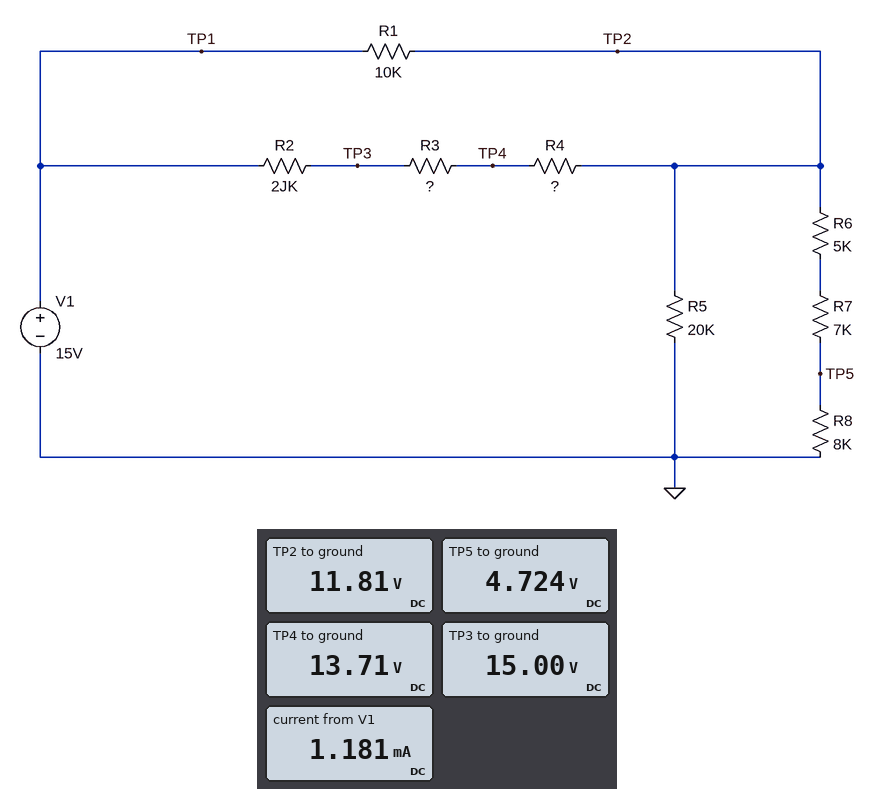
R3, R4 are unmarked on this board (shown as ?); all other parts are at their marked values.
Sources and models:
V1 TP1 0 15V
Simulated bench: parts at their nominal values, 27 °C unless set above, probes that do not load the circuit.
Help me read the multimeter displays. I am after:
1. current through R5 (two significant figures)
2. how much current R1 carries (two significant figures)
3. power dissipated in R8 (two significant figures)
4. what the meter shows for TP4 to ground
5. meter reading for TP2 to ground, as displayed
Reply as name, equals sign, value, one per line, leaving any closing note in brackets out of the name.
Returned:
current through R5 = 590 µA
how much current R1 carries = 320 µA
power dissipated in R8 = 2.8 mW
what the meter shows for TP4 to ground = 13.71 V
meter reading for TP2 to ground, as displayed = 11.81 V
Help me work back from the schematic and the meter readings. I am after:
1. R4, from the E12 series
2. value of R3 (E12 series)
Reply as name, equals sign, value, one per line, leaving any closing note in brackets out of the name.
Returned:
R4, from the E12 series = 2.2 kΩ
value of R3 = 1.5 kΩ
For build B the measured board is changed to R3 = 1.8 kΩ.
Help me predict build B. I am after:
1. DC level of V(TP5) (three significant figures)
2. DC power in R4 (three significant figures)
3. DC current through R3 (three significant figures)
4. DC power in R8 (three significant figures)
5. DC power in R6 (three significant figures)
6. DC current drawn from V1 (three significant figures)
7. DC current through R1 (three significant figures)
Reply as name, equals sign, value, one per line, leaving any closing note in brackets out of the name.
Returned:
DC level of V(TP5) = 4.67 V
DC power in R4 = 1.53 mW
DC current through R3 = 833 µA
DC power in R8 = 2.72 mW
DC power in R6 = 1.70 mW
DC current drawn from V1 = 1.17 mA
DC current through R1 = 333 µA
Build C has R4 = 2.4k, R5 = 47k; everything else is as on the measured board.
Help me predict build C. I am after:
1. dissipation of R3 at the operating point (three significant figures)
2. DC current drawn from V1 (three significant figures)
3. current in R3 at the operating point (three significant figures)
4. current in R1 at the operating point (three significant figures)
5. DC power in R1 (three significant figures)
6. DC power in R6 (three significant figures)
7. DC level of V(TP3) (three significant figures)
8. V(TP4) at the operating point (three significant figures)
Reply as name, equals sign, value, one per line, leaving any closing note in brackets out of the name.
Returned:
dissipation of R3 at the operating point = 616 µW
DC current drawn from V1 = 891 µA
current in R3 at the operating point = 641 µA
current in R1 at the operating point = 250 µA
DC power in R1 = 625 µW
DC power in R6 = 1.95 mW
DC level of V(TP3) = 15.0 V
V(TP4) at the operating point = 14.0 V
